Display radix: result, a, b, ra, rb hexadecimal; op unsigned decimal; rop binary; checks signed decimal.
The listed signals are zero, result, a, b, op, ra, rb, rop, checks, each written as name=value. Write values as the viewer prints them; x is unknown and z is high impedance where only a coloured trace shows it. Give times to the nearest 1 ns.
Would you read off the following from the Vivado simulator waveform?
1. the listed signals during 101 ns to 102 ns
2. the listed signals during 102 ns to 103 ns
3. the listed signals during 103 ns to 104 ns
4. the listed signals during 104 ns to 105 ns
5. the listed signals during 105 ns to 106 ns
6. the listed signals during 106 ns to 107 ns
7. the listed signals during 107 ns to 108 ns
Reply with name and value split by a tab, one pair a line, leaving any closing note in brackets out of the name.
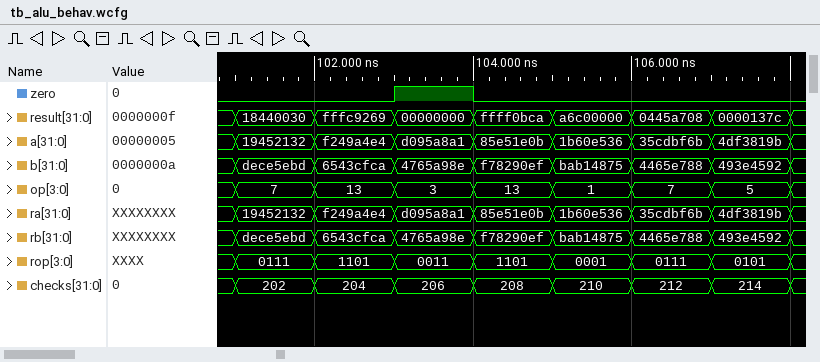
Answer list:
the listed signals during 101 ns to 102 ns	zero=0, result=18440030, a=19452132, b=dece5ebd, op=7, ra=19452132, rb=dece5ebd, rop=0111, checks=202
the listed signals during 102 ns to 103 ns	zero=0, result=fffc9269, a=f249a4e4, b=6543cfca, op=13, ra=f249a4e4, rb=6543cfca, rop=1101, checks=204
the listed signals during 103 ns to 104 ns	zero=1, result=00000000, a=d095a8a1, b=4765a98e, op=3, ra=d095a8a1, rb=4765a98e, rop=0011, checks=206
the listed signals during 104 ns to 105 ns	zero=0, result=ffff0bca, a=85e51e0b, b=f78290ef, op=13, ra=85e51e0b, rb=f78290ef, rop=1101, checks=208
the listed signals during 105 ns to 106 ns	zero=0, result=a6c00000, a=1b60e536, b=bab14875, op=1, ra=1b60e536, rb=bab14875, rop=0001, checks=210
the listed signals during 106 ns to 107 ns	zero=0, result=0445a708, a=35cdbf6b, b=4465e788, op=7, ra=35cdbf6b, rb=4465e788, rop=0111, checks=212
the listed signals during 107 ns to 108 ns	zero=0, result=0000137c, a=4df3819b, b=493e4592, op=5, ra=4df3819b, rb=493e4592, rop=0101, checks=214
